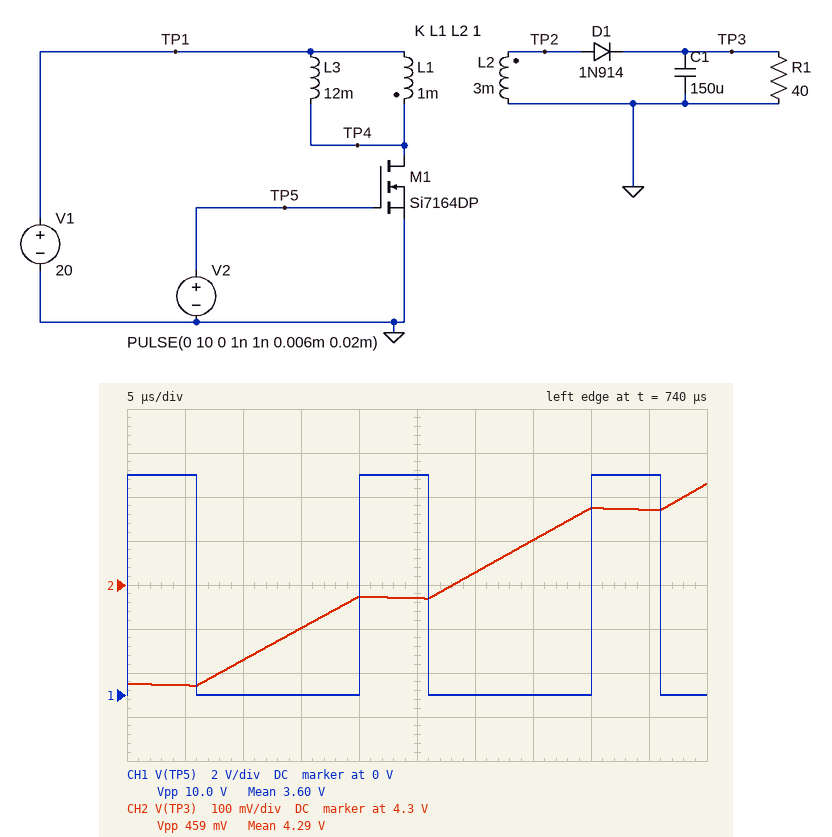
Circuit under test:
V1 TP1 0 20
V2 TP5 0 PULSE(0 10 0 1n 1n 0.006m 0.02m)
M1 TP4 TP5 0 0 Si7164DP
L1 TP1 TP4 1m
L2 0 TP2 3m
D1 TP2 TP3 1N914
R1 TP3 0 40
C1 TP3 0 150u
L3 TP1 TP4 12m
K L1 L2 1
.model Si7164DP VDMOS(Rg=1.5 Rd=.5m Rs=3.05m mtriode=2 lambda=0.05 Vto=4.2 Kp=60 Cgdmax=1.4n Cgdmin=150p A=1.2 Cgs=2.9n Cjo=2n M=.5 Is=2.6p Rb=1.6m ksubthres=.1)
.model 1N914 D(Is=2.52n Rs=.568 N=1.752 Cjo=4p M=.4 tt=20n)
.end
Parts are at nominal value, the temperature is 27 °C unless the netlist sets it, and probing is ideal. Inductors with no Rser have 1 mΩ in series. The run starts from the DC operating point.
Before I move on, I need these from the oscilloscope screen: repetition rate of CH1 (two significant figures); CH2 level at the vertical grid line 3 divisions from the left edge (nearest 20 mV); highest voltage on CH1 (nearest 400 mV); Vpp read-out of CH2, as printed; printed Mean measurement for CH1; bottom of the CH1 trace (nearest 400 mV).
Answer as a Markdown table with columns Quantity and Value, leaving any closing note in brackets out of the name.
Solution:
| Quantity | Value |
|---|---|
| repetition rate of CH1 | 50 kHz |
| CH2 level at the vertical grid line 3 divisions from the left edge | 4.20 V |
| highest voltage on CH1 | 10.0 V |
| Vpp read-out of CH2, as printed | 459 mV |
| printed Mean measurement for CH1 | 3.60 V |
| bottom of the CH1 trace | 0 V |
